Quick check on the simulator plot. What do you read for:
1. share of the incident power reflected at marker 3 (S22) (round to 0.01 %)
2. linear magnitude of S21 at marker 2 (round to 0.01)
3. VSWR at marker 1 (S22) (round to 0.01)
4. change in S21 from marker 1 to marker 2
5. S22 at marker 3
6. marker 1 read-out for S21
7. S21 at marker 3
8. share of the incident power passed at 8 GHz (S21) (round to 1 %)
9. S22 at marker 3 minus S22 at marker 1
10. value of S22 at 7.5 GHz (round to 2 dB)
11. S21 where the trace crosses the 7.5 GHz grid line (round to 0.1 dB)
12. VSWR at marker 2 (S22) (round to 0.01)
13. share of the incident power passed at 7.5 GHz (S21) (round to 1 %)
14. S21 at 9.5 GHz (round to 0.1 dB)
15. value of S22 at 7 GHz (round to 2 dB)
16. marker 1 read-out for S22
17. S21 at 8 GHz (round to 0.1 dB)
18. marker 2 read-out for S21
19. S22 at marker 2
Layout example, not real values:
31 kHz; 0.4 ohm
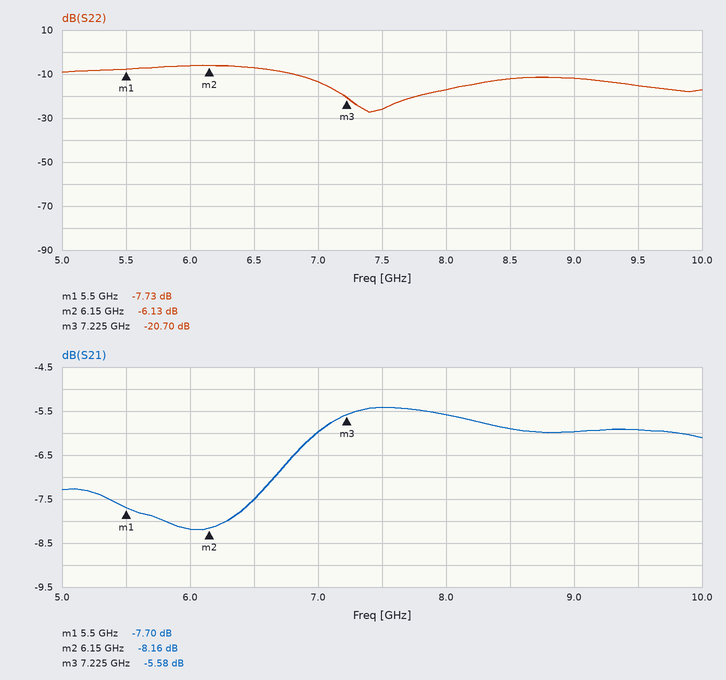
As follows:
0.85 %; 0.39; 2.39; -0.46 dB; -20.70 dB; -7.70 dB; -5.58 dB; 28 %; -12.97 dB; -26 dB; -5.4 dB; 2.95; 29 %; -5.9 dB; -14 dB; -7.73 dB; -5.6 dB; -8.16 dB; -6.13 dB
